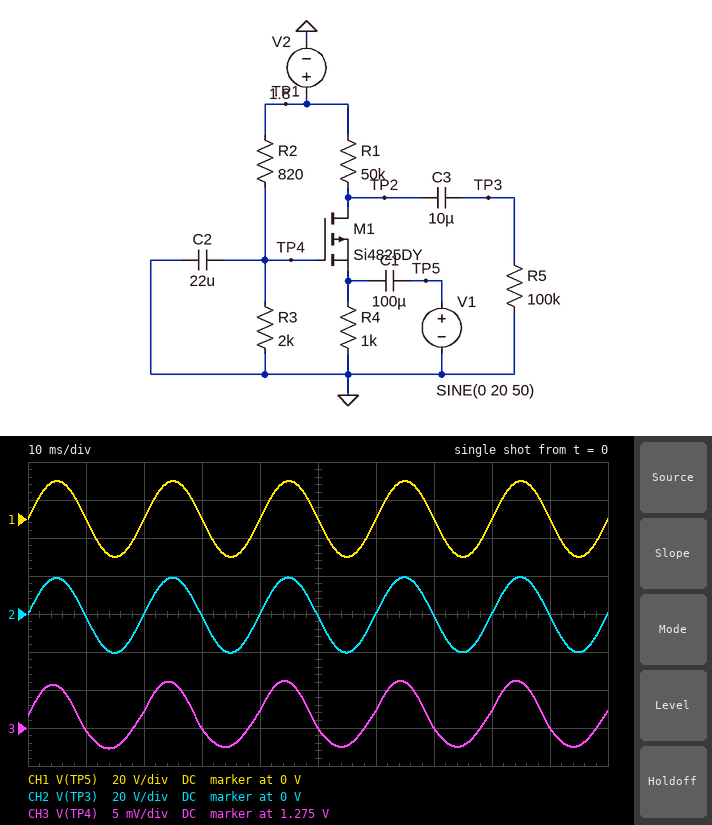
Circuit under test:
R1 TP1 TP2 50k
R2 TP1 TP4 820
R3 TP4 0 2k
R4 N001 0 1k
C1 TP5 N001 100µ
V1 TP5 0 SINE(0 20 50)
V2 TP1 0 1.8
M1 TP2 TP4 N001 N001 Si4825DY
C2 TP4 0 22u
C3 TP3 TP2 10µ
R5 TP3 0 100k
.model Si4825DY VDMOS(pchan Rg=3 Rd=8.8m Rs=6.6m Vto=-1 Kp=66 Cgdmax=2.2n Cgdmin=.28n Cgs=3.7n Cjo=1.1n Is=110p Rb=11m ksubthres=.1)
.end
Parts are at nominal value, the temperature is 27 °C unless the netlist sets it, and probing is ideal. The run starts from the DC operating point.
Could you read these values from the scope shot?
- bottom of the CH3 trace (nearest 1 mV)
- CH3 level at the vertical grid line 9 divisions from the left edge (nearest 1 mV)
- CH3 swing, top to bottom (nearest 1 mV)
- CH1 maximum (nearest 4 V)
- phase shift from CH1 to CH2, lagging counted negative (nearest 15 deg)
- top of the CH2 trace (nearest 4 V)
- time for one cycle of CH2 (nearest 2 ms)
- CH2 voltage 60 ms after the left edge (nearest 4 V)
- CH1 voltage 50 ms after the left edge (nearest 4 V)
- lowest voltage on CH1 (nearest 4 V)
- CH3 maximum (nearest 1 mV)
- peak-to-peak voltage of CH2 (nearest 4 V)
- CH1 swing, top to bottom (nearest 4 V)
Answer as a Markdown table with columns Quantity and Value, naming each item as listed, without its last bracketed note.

| Quantity | Value |
|---|---|
| bottom of the CH3 trace | 1.272 V |
| CH3 level at the vertical grid line 9 divisions from the left edge | 1.275 V |
| CH3 swing, top to bottom | 9 mV |
| CH1 maximum | 20 V |
| phase shift from CH1 to CH2, lagging counted negative | 0 deg |
| top of the CH2 trace | 20 V |
| time for one cycle of CH2 | 20 ms |
| CH2 voltage 60 ms after the left edge | 0 V |
| CH1 voltage 50 ms after the left edge | 0 V |
| lowest voltage on CH1 | -20 V |
| CH3 maximum | 1.281 V |
| peak-to-peak voltage of CH2 | 40 V |
| CH1 swing, top to bottom | 40 V |
